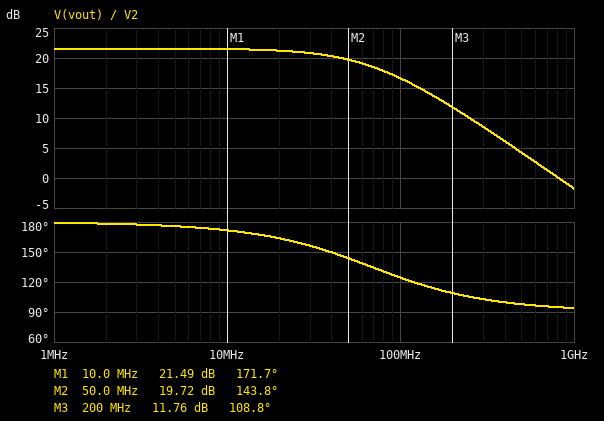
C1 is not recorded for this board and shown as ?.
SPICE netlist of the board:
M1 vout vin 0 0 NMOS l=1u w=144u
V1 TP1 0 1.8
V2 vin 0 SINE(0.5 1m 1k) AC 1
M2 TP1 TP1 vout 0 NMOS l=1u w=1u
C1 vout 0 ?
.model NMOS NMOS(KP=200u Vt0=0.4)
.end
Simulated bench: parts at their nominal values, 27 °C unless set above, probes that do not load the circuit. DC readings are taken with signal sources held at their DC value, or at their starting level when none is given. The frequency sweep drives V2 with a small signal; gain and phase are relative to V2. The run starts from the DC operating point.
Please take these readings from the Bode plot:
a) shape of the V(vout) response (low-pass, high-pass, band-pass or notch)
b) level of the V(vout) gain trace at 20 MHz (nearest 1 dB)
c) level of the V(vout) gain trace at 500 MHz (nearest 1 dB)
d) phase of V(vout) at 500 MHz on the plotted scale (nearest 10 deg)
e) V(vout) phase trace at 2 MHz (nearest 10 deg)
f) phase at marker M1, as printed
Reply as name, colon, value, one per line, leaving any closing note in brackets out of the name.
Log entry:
shape of the V(vout) response: low-pass
level of the V(vout) gain trace at 20 MHz: 21 dB
level of the V(vout) gain trace at 500 MHz: 4 dB
phase of V(vout) at 500 MHz on the plotted scale: 100 deg
V(vout) phase trace at 2 MHz: 180 deg
phase at marker M1, as printed: 171.7 deg
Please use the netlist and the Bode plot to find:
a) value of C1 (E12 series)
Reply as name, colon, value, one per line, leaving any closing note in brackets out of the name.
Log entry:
value of C1: 560 fF
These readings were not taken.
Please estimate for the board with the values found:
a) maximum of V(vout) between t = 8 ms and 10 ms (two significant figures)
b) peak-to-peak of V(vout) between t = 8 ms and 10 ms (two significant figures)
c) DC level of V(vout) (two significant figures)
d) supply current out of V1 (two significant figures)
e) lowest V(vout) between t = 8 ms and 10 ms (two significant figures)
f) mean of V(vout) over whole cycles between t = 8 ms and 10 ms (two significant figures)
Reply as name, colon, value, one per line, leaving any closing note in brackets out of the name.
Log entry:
maximum of V(vout) between t = 8 ms and 10 ms: 210 mV
peak-to-peak of V(vout) between t = 8 ms and 10 ms: 24 mV
DC level of V(vout): 200 mV
supply current out of V1: 140 µA
lowest V(vout) between t = 8 ms and 10 ms: 190 mV
mean of V(vout) over whole cycles between t = 8 ms and 10 ms: 200 mV
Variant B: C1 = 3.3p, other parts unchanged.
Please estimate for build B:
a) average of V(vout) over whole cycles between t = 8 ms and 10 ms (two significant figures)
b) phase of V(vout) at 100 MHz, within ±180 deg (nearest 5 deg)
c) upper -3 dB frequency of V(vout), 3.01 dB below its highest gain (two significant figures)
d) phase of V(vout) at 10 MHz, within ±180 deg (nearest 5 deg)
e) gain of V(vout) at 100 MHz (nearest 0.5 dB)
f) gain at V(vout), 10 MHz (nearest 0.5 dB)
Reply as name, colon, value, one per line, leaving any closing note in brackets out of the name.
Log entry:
average of V(vout) over whole cycles between t = 8 ms and 10 ms: 200 mV
phase of V(vout) at 100 MHz, within ±180 deg: 95 deg
upper -3 dB frequency of V(vout), 3.01 dB below its highest gain: 12 MHz
phase of V(vout) at 10 MHz, within ±180 deg: 140 deg
gain of V(vout) at 100 MHz: 3.0 dB
gain at V(vout), 10 MHz: 19.0 dB
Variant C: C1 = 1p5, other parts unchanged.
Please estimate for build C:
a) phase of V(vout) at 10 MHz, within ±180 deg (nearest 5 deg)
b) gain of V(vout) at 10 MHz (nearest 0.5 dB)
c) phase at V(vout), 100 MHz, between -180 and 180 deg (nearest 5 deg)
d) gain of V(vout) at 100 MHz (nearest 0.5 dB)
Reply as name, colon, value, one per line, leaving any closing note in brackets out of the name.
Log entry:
phase of V(vout) at 10 MHz, within ±180 deg: 160 deg
gain of V(vout) at 10 MHz: 21.0 dB
phase at V(vout), 100 MHz, between -180 and 180 deg: 105 deg
gain of V(vout) at 100 MHz: 9.5 dB
